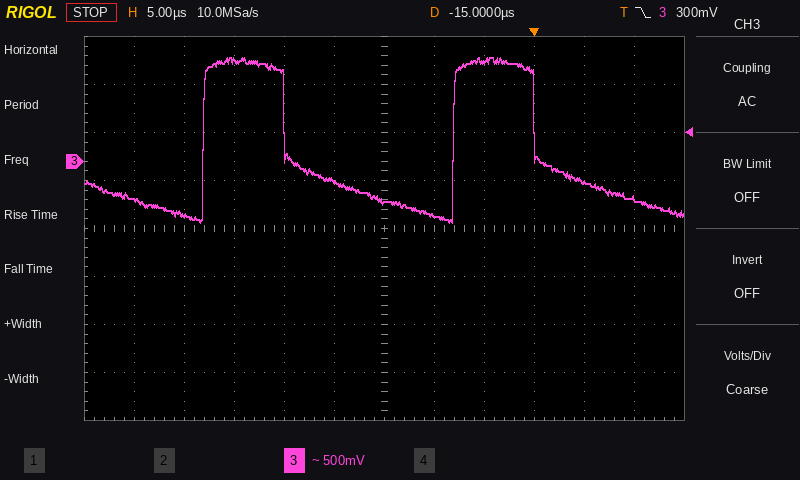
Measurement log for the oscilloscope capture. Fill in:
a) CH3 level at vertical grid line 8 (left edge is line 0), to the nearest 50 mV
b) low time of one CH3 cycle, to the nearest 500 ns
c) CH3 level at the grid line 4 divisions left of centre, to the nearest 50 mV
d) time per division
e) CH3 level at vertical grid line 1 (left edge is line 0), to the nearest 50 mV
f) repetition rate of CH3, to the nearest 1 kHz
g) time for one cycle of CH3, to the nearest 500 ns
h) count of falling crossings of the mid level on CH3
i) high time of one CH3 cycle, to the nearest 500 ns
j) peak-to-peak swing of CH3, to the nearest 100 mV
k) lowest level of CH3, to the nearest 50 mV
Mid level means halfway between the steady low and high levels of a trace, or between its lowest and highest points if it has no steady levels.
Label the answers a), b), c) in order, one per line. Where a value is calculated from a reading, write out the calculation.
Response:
a) 1.05 V
b) 17.0 µs
c) -550 mV
d) 5 µs
e) -400 mV
f) 1 / 25.0 µs ≈ 40 kHz
g) 25.0 µs
h) 2
i) 8.0 µs
j) 1.70 V
k) -650 mV
